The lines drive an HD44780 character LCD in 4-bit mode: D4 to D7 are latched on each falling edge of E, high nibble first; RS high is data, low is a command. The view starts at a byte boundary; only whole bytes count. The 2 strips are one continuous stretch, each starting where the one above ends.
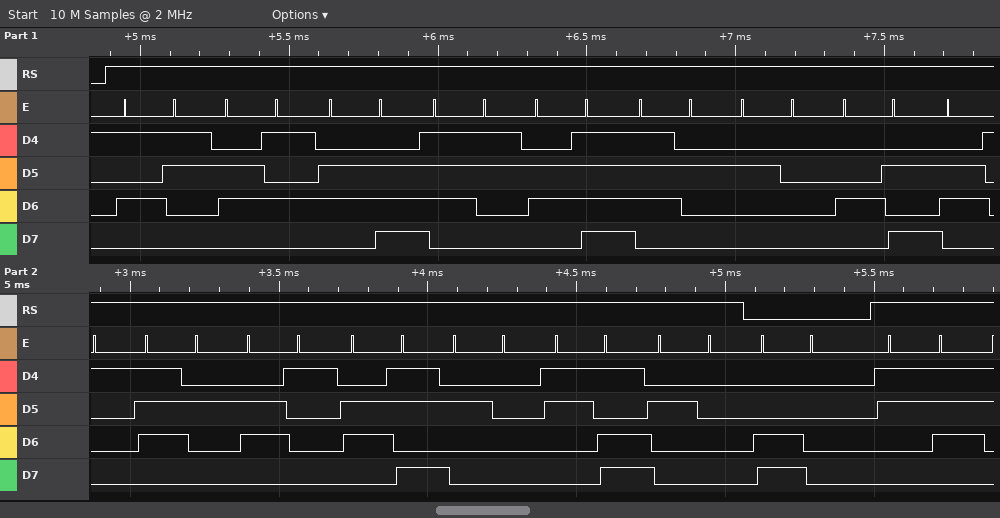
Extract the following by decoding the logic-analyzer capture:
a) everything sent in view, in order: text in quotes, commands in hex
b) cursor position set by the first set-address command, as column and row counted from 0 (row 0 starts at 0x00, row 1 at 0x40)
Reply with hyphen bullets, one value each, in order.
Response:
- "Sensor Jarak = " 0xC0 "7"
- column 0, row 1
